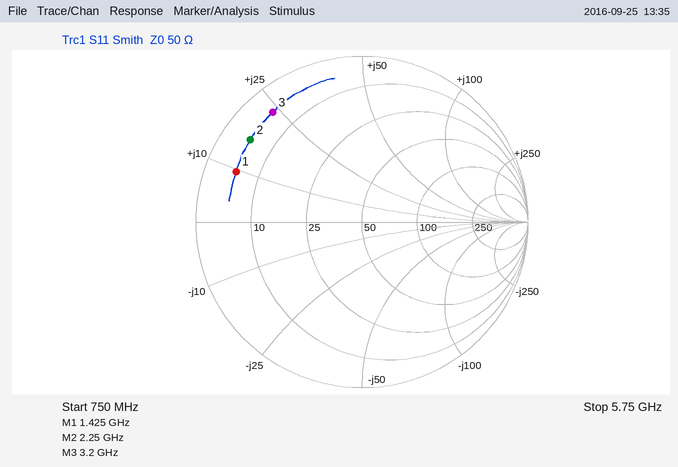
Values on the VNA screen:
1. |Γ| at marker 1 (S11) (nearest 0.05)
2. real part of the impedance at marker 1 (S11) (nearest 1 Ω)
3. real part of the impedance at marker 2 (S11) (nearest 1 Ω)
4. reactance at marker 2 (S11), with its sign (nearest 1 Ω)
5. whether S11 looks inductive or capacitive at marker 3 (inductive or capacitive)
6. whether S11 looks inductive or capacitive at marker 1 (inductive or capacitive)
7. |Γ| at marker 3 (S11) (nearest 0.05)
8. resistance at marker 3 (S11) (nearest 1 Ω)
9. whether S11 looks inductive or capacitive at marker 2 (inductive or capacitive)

0.80
5 Ω
5 Ω
+16 Ω
inductive
inductive
0.85
5 Ω
inductive
